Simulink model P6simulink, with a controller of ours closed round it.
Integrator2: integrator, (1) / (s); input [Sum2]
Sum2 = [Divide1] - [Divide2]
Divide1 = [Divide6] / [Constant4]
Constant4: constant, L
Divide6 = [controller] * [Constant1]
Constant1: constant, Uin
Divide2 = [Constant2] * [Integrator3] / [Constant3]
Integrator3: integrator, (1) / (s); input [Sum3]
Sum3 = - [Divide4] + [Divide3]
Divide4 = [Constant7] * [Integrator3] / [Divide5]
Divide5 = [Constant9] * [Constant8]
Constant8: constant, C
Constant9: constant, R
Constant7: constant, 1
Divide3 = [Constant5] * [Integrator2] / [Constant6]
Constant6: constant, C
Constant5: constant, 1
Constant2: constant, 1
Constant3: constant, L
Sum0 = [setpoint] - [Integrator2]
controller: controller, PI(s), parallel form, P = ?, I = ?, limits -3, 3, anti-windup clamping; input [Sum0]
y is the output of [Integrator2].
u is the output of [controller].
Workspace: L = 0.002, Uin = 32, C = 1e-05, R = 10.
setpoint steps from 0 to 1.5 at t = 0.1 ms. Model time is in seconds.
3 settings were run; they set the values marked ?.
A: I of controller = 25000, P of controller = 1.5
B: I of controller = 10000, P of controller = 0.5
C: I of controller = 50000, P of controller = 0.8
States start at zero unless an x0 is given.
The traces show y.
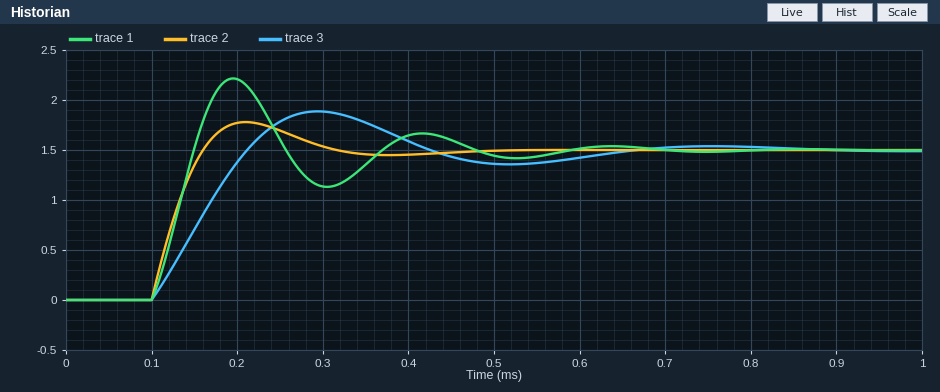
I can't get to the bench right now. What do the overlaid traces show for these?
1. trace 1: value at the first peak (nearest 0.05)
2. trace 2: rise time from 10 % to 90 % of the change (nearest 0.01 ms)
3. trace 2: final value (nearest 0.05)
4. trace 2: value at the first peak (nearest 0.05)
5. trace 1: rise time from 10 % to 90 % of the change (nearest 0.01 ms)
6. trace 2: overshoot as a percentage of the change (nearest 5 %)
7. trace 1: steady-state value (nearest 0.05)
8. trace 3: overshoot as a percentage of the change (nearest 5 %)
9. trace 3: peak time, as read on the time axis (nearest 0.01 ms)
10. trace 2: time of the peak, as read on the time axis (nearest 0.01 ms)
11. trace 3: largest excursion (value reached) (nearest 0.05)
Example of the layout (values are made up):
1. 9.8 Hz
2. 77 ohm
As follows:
1. 2.20
2. 0.05 ms
3. 1.50
4. 1.80
5. 0.04 ms
6. 20 %
7. 1.50
8. 25 %
9. 0.29 ms
10. 0.21 ms
11. 1.90
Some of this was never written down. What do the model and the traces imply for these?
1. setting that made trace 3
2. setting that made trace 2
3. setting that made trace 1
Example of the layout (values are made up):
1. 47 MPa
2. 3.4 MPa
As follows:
1. B
2. A
3. C
